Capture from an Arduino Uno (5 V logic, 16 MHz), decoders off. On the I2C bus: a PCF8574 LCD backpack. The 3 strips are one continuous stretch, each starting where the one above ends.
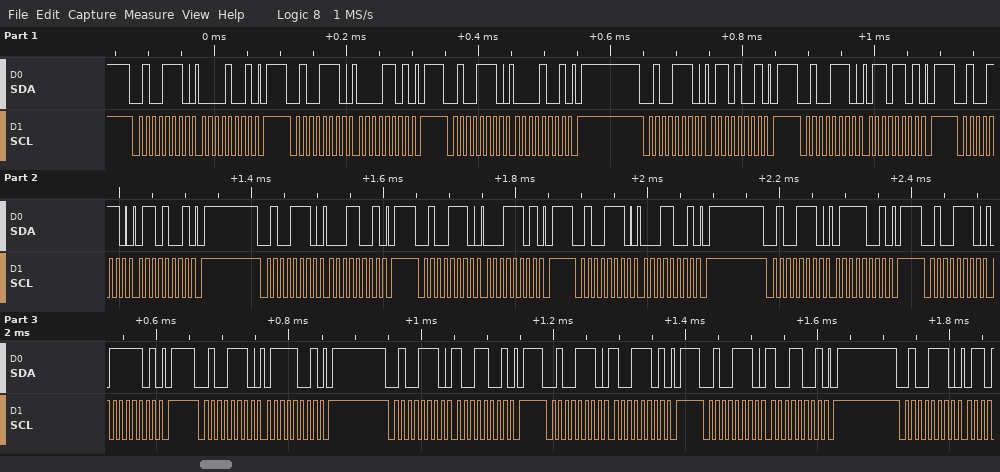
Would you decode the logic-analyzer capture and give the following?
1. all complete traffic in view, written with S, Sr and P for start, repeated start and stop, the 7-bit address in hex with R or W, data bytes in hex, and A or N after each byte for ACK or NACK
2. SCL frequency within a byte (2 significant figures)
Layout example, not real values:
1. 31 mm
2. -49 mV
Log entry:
1. S 27W A 09 A P S 27W A 0D A P S 27W A 09 A P S 27W A 69 A P S 27W A 6D A P S 27W A 69 A P S 27W A 19 A P S 27W A 1D A P S 27W A 19 A P S 27W A 79 A P S 27W A 7D A P S 27W A 79 A P S 27W A 99 A P S 27W A 9D A P S 27W A 99 A P S 27W A
2. 100 kHz
